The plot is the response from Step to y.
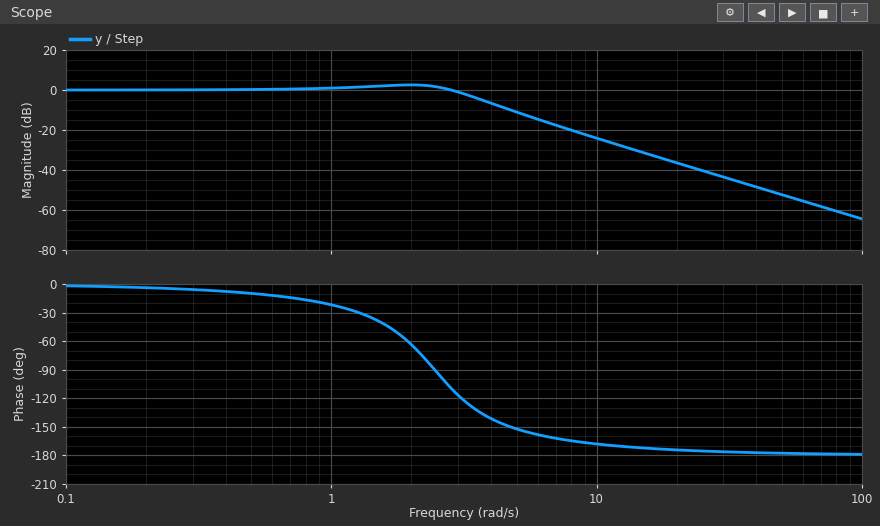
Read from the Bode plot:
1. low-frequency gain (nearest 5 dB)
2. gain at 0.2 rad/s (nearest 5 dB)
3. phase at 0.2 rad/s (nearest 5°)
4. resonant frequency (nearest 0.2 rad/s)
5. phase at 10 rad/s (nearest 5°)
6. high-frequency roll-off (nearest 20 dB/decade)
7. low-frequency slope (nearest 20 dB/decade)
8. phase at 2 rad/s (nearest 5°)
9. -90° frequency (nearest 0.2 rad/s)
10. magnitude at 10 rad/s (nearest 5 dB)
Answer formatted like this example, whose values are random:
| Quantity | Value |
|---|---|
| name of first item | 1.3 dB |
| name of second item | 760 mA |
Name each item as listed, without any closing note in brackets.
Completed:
| Quantity | Value |
|---|---|
| low-frequency gain | 0 dB |
| gain at 0.2 rad/s | 0 dB |
| phase at 0.2 rad/s | -5° |
| resonant frequency | 2.0 rad/s |
| phase at 10 rad/s | -170° |
| high-frequency roll-off | -40 dB/decade |
| low-frequency slope | 0 dB/decade |
| phase at 2 rad/s | -65° |
| -90° frequency | 2.4 rad/s |
| magnitude at 10 rad/s | -25 dB |
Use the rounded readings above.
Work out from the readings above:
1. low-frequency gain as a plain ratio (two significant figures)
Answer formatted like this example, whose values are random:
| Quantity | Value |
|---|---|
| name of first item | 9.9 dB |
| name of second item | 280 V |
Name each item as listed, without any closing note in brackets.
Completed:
| Quantity | Value |
|---|---|
| low-frequency gain as a plain ratio | 1.0 |
